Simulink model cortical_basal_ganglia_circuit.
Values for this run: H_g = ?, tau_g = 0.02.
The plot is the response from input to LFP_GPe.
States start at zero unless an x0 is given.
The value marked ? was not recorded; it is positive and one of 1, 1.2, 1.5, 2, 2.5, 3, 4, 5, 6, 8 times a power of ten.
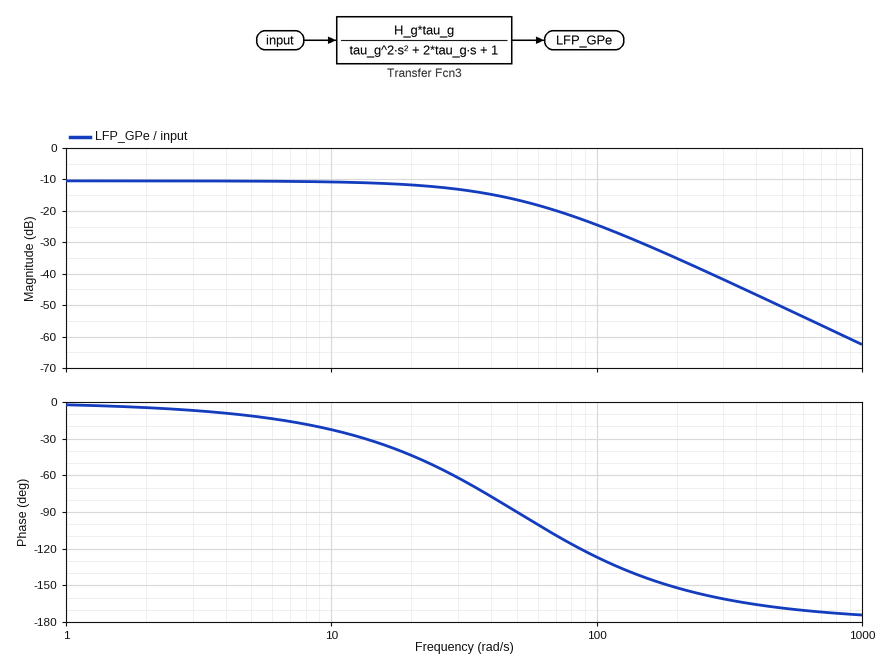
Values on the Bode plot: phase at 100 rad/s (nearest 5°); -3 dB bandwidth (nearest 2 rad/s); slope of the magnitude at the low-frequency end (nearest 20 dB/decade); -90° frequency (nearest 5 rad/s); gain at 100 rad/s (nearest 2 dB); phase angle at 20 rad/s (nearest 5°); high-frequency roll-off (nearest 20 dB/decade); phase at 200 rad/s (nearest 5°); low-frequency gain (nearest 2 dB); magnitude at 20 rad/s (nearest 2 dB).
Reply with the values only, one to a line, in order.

-125°
32 rad/s
0 dB/decade
50 rad/s
-24 dB
-45°
-40 dB/decade
-150°
-10 dB
-12 dB
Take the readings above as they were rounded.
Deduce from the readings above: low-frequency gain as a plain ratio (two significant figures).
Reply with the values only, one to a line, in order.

0.32
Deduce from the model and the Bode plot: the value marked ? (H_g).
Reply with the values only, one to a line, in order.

15
